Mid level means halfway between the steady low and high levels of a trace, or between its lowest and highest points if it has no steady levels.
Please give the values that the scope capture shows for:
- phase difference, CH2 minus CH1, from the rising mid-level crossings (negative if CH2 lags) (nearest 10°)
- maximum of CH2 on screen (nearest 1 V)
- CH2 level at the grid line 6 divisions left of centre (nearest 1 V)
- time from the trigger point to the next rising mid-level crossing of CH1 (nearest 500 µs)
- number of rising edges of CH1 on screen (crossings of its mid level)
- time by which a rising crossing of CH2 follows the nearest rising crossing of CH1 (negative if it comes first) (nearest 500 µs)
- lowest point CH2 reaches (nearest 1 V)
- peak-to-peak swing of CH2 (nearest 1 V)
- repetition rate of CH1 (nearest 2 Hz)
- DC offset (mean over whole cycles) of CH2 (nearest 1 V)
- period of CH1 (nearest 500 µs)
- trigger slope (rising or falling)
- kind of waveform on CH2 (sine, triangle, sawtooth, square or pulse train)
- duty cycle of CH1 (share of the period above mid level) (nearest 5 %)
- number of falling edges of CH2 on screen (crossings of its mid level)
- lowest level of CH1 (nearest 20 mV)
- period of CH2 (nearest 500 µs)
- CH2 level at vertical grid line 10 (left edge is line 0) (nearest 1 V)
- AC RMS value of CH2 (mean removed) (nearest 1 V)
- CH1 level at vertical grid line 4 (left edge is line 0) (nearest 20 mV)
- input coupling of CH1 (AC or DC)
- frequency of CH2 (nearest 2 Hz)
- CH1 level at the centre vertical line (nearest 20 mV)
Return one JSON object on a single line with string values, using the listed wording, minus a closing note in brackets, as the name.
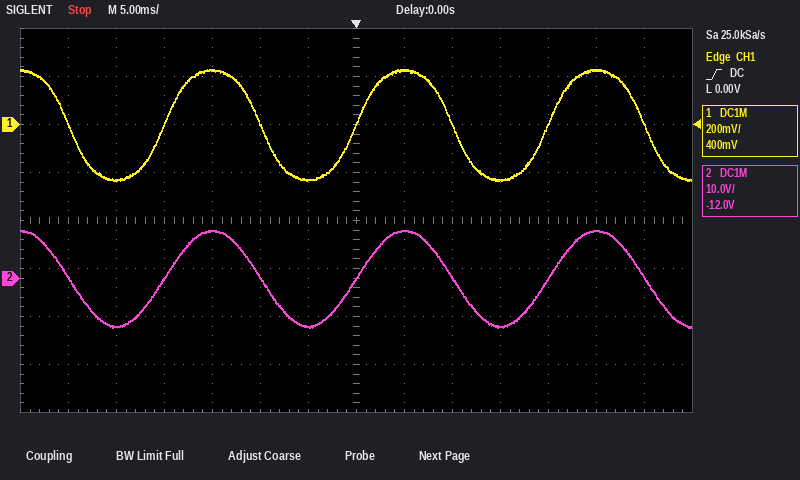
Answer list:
{"phase difference, CH2 minus CH1, from the rising mid-level crossings (negative if CH2 lags)": "0°", "maximum of CH2 on screen": "10 V", "CH2 level at the grid line 6 divisions left of centre": "0 V", "time from the trigger point to the next rising mid-level crossing of CH1": "20.0 ms", "number of rising edges of CH1 on screen": "3", "time by which a rising crossing of CH2 follows the nearest rising crossing of CH1 (negative if it comes first)": "0.0 ms", "lowest point CH2 reaches": "-10 V", "peak-to-peak swing of CH2": "20 V", "repetition rate of CH1": "50 Hz", "DC offset (mean over whole cycles) of CH2": "0 V", "period of CH1": "20.0 ms", "trigger slope": "rising", "kind of waveform on CH2": "sine", "duty cycle of CH1 (share of the period above mid level)": "50 %", "number of falling edges of CH2 on screen": "4", "lowest level of CH1": "-240 mV", "period of CH2": "20.0 ms", "CH2 level at vertical grid line 10 (left edge is line 0)": "-10 V", "AC RMS value of CH2 (mean removed)": "7 V", "CH1 level at vertical grid line 4 (left edge is line 0)": "220 mV", "input coupling of CH1": "DC", "frequency of CH2": "50 Hz", "CH1 level at the centre vertical line": "0 mV"}
